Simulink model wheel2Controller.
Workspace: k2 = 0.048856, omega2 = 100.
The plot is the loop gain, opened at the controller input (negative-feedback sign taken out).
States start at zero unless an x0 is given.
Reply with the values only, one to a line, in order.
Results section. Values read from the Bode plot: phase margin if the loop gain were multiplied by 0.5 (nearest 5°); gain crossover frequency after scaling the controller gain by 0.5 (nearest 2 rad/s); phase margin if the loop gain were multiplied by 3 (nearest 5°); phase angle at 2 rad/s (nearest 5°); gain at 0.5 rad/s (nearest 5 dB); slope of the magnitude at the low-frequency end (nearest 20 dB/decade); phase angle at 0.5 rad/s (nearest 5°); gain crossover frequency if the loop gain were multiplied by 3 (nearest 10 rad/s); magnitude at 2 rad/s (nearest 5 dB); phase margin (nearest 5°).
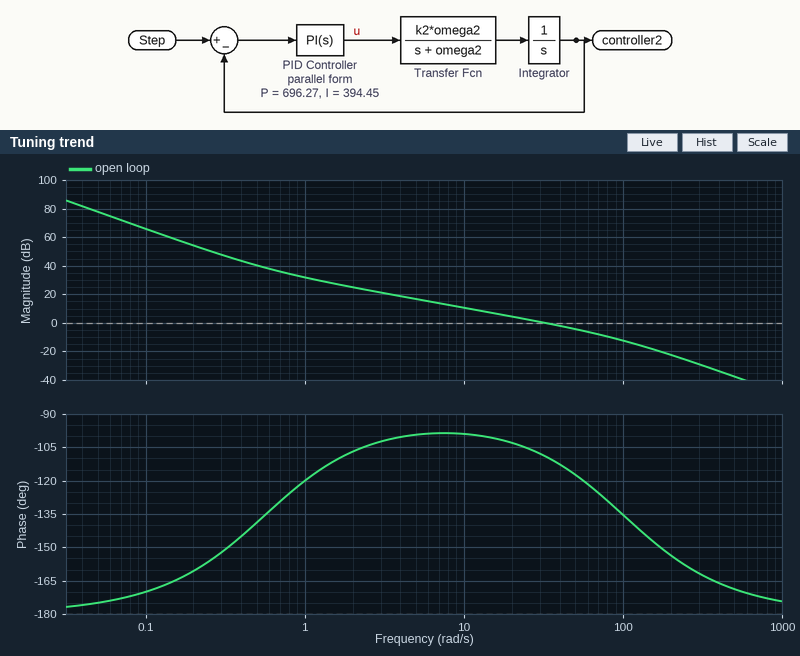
80°
16 rad/s
50°
-105°
40 dB
-40 dB/decade
-140°
80 rad/s
25 dB
70°
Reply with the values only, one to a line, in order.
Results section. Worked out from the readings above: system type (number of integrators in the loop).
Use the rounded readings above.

2
